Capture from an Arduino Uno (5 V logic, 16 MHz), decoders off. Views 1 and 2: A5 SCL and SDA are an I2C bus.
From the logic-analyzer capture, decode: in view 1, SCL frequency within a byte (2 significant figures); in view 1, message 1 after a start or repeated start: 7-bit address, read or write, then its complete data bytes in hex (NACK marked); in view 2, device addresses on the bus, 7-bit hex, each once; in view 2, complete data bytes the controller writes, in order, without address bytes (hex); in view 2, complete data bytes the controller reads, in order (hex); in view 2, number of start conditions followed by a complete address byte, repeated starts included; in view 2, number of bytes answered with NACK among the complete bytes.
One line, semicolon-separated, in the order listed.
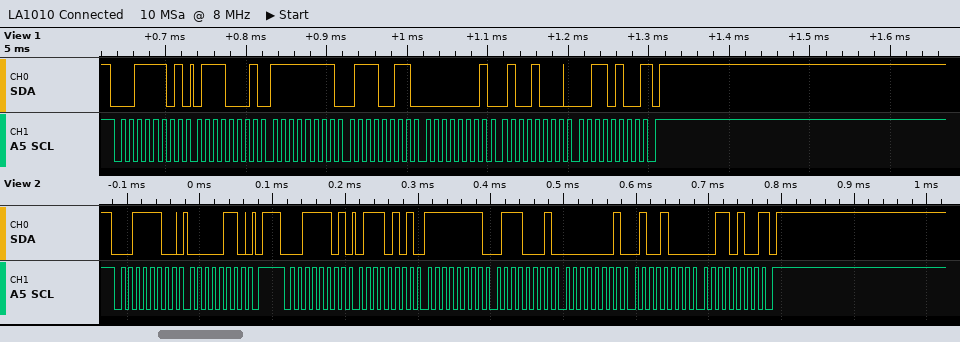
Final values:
100 kHz; 0x1E read: 71 FF 73 01 48 34 NACK; 0x1E; 06; 75 FF 71 01 48 34; 2; 1
